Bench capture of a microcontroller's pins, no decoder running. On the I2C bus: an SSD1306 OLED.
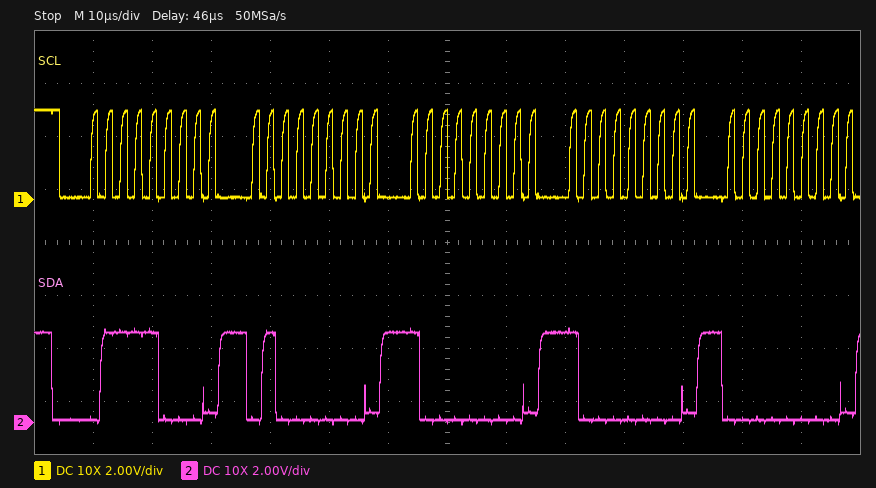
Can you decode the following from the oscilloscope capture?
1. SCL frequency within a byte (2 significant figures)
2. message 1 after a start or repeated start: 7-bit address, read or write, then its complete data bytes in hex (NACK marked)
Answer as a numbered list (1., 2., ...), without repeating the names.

1. 400 kHz
2. 0x3C write: 40 80 80 00
